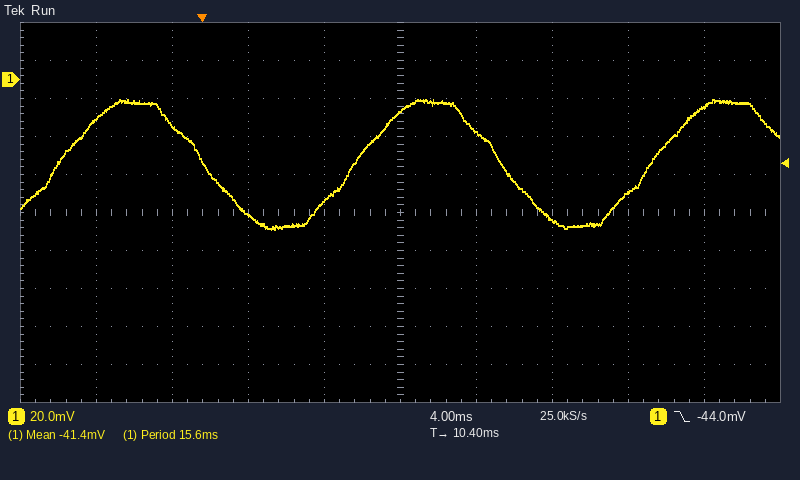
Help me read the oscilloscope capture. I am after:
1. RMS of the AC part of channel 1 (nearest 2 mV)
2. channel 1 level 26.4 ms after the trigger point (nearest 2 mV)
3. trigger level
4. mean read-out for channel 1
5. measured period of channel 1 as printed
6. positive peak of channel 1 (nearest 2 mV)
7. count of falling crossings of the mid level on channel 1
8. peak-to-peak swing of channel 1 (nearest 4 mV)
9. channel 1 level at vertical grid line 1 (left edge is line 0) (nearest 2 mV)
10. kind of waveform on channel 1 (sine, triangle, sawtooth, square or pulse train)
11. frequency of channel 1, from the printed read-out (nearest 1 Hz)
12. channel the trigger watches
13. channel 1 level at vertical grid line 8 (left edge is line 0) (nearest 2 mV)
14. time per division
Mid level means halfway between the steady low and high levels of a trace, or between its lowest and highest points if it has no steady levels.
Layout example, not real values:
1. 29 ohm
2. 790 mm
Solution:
1. 24 mV
2. -14 mV
3. -44.0 mV
4. -41.4 mV
5. 15.6 ms
6. -10 mV
7. 2
8. 68 mV
9. -20 mV
10. sine
11. 64 Hz
12. channel 1
13. -60 mV
14. 4 ms
